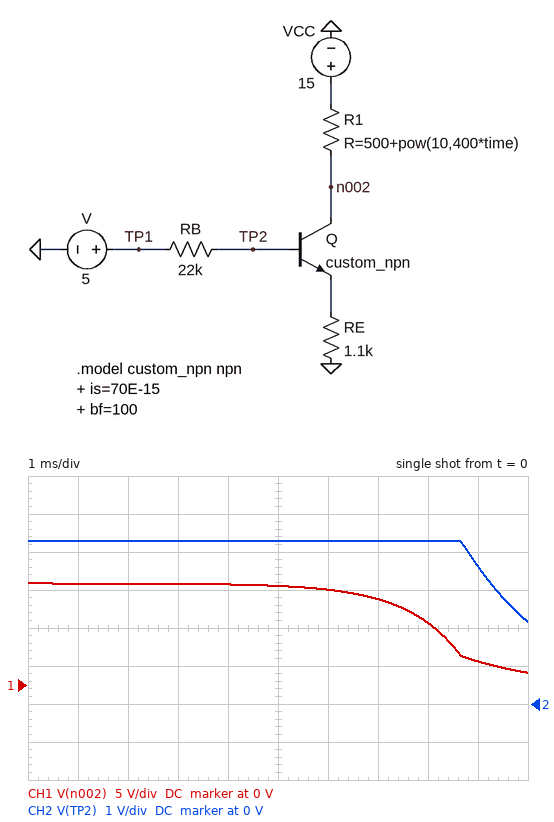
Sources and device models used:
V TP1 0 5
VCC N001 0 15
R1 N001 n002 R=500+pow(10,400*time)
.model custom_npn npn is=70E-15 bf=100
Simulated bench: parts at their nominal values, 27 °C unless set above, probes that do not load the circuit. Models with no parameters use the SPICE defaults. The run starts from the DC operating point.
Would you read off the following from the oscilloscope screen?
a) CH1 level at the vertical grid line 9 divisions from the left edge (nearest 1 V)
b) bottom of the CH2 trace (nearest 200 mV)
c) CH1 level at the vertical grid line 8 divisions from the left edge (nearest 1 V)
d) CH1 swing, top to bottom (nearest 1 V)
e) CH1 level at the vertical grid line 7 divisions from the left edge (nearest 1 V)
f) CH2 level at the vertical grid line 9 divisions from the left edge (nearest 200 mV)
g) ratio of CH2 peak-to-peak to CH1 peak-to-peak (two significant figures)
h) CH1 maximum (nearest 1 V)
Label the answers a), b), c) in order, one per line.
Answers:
a) 3 V
b) 2.2 V
c) 8 V
d) 12 V
e) 11 V
f) 3.6 V
g) 0.18
h) 13 V
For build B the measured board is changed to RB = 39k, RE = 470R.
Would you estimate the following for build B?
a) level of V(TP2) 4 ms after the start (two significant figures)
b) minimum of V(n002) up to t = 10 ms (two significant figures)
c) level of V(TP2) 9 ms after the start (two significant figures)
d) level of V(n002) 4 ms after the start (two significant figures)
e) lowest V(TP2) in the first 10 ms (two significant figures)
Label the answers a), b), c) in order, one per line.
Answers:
a) 3.0 V
b) 760 mV
c) 2.1 V
d) 12 V
e) 1.3 V
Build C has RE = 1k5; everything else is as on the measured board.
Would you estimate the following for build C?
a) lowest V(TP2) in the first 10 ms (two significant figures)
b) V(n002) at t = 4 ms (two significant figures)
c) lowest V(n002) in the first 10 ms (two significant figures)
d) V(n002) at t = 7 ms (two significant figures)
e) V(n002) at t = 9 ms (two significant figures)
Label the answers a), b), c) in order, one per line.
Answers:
a) 2.6 V
b) 14 V
c) 2.1 V
d) 12 V
e) 3.9 V
